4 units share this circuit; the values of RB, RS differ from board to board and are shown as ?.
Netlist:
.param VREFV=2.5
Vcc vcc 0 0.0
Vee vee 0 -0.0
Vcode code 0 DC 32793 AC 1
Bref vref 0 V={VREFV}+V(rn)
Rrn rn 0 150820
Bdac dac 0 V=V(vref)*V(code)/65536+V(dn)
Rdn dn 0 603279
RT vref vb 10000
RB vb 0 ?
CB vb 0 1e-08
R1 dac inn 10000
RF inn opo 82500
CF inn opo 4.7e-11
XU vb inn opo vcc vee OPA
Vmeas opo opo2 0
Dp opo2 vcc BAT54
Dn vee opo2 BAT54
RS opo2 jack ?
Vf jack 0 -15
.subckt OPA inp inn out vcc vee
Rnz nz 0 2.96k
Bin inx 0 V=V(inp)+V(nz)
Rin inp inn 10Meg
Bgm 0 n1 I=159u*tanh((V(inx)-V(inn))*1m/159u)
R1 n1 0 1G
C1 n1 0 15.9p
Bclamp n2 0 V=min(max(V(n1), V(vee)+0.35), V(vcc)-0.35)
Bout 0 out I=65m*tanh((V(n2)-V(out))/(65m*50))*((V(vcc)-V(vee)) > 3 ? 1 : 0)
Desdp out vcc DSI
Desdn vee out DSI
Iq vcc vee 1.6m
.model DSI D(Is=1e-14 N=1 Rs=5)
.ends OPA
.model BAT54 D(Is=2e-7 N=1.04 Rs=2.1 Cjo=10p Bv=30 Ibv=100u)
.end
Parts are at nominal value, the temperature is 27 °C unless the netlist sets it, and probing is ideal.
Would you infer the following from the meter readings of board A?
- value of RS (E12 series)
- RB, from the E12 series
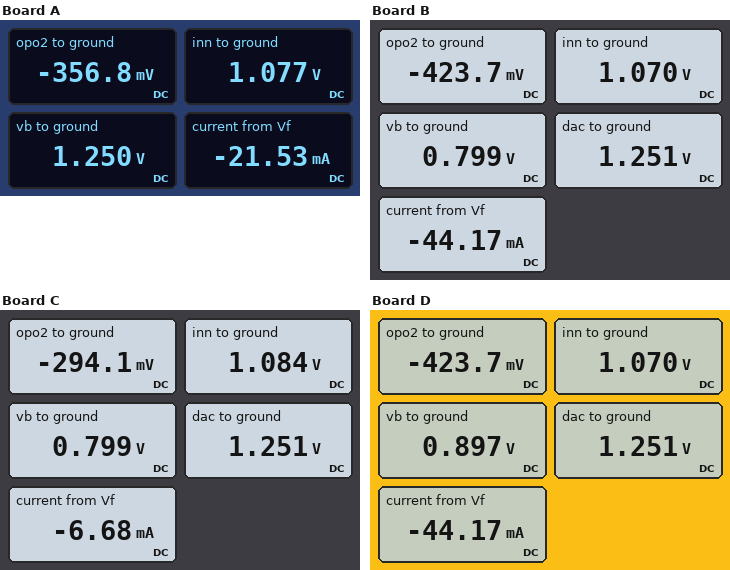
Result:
680 Ω
10 kΩ
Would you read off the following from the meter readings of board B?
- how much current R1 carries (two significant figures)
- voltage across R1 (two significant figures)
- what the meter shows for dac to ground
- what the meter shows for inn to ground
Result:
18 µA
180 mV
1.251 V
1.070 V
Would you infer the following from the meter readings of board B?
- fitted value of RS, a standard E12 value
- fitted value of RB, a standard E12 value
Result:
330 Ω
4.7 kΩ
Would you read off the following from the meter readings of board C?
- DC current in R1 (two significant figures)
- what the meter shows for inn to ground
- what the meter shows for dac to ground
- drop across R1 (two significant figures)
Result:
17 µA
1.084 V
1.251 V
170 mV
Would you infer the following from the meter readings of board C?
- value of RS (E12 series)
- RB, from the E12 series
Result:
2.2 kΩ
4.7 kΩ
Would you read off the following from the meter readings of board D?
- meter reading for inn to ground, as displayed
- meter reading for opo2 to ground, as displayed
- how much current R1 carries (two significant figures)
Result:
1.070 V
-423.7 mV
18 µA
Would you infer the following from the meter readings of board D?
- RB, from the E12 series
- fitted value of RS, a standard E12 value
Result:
5.6 kΩ
330 Ω
